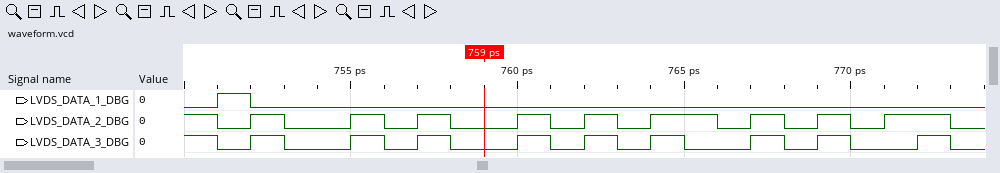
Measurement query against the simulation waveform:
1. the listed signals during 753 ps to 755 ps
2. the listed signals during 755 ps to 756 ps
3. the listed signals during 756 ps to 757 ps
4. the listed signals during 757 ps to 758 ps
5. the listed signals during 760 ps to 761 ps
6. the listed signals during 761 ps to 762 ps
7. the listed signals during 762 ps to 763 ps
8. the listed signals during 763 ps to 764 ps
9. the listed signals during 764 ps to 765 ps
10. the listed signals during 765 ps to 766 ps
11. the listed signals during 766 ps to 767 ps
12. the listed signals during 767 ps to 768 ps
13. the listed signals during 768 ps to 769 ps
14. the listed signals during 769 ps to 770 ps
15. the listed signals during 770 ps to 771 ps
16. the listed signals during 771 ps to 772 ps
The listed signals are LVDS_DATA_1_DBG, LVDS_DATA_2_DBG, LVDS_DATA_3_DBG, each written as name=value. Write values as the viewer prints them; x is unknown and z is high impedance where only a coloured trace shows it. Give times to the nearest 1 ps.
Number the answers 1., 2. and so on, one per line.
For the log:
1. LVDS_DATA_1_DBG=0, LVDS_DATA_2_DBG=0, LVDS_DATA_3_DBG=0
2. LVDS_DATA_1_DBG=0, LVDS_DATA_2_DBG=1, LVDS_DATA_3_DBG=1
3. LVDS_DATA_1_DBG=0, LVDS_DATA_2_DBG=0, LVDS_DATA_3_DBG=0
4. LVDS_DATA_1_DBG=0, LVDS_DATA_2_DBG=1, LVDS_DATA_3_DBG=1
5. LVDS_DATA_1_DBG=0, LVDS_DATA_2_DBG=1, LVDS_DATA_3_DBG=1
6. LVDS_DATA_1_DBG=0, LVDS_DATA_2_DBG=0, LVDS_DATA_3_DBG=0
7. LVDS_DATA_1_DBG=0, LVDS_DATA_2_DBG=1, LVDS_DATA_3_DBG=1
8. LVDS_DATA_1_DBG=0, LVDS_DATA_2_DBG=0, LVDS_DATA_3_DBG=0
9. LVDS_DATA_1_DBG=0, LVDS_DATA_2_DBG=1, LVDS_DATA_3_DBG=1
10. LVDS_DATA_1_DBG=0, LVDS_DATA_2_DBG=1, LVDS_DATA_3_DBG=0
11. LVDS_DATA_1_DBG=0, LVDS_DATA_2_DBG=0, LVDS_DATA_3_DBG=0
12. LVDS_DATA_1_DBG=0, LVDS_DATA_2_DBG=1, LVDS_DATA_3_DBG=1
13. LVDS_DATA_1_DBG=0, LVDS_DATA_2_DBG=0, LVDS_DATA_3_DBG=0
14. LVDS_DATA_1_DBG=0, LVDS_DATA_2_DBG=1, LVDS_DATA_3_DBG=1
15. LVDS_DATA_1_DBG=0, LVDS_DATA_2_DBG=0, LVDS_DATA_3_DBG=0
16. LVDS_DATA_1_DBG=0, LVDS_DATA_2_DBG=1, LVDS_DATA_3_DBG=0
